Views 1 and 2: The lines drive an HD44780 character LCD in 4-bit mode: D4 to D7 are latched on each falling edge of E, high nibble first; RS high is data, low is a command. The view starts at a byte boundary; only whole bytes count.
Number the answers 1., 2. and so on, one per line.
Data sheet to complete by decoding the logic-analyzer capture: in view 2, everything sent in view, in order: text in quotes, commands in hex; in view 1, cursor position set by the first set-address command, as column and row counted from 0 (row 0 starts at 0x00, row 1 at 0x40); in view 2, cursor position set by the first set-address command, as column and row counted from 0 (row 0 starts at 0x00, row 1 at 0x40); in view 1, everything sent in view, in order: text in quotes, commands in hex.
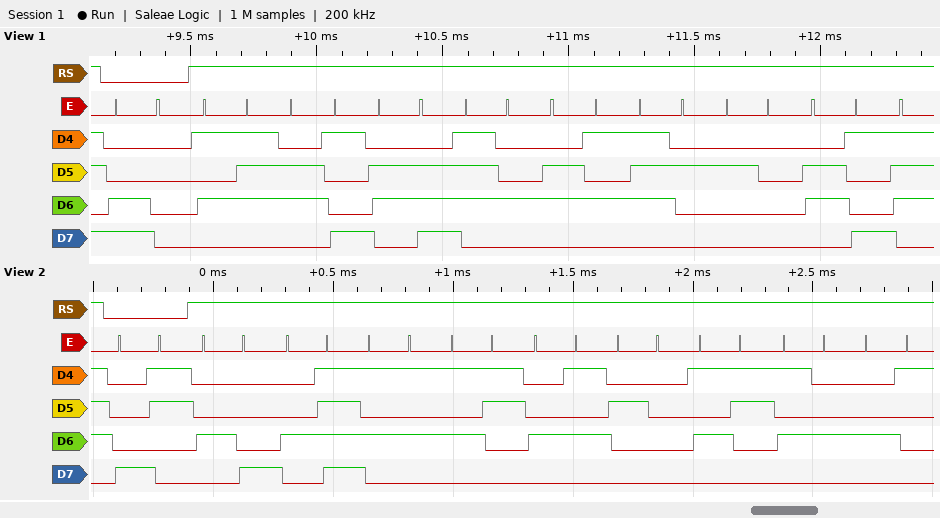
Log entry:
1. 0x83 "HOUSE STA"
2. column 0, row 1
3. column 3, row 0
4. 0xC0 "Winter i"
